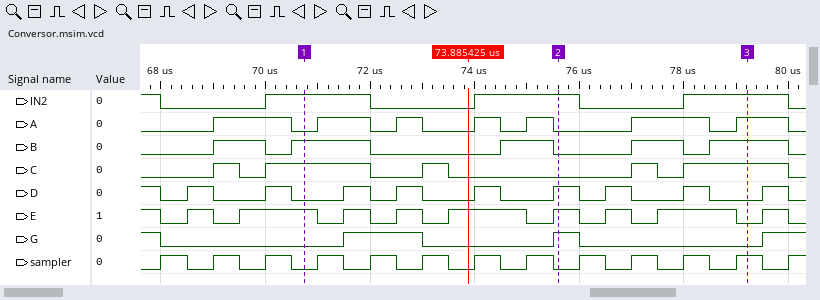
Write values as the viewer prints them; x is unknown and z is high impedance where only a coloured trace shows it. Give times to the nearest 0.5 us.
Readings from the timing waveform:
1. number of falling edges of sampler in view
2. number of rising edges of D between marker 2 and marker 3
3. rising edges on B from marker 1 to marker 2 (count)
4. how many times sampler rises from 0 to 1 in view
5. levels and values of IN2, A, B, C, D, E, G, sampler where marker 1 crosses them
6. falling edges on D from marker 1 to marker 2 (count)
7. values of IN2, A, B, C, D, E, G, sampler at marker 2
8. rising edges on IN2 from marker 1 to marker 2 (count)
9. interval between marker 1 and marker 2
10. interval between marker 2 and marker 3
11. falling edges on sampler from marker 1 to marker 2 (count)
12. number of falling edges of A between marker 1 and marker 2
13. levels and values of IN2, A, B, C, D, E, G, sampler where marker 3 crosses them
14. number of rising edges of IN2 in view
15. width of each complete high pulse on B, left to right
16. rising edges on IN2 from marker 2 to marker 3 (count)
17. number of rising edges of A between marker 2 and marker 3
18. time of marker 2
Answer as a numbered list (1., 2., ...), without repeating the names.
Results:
1. 12
2. 2
3. 1
4. 13
5. IN2=1, A=0, B=1, C=1, D=0, E=1, G=0, sampler=0
6. 3
7. IN2=1, A=0, B=0, C=0, D=1, E=1, G=1, sampler=0
8. 1
9. 5 us
10. 3.5 us
11. 5
12. 4
13. IN2=1, A=1, B=1, C=1, D=0, E=0, G=0, sampler=1
14. 3
15. 1 us, 1.5 us, 1 us, 1 us, 1.5 us
16. 1
17. 2
18. 75.5 us
